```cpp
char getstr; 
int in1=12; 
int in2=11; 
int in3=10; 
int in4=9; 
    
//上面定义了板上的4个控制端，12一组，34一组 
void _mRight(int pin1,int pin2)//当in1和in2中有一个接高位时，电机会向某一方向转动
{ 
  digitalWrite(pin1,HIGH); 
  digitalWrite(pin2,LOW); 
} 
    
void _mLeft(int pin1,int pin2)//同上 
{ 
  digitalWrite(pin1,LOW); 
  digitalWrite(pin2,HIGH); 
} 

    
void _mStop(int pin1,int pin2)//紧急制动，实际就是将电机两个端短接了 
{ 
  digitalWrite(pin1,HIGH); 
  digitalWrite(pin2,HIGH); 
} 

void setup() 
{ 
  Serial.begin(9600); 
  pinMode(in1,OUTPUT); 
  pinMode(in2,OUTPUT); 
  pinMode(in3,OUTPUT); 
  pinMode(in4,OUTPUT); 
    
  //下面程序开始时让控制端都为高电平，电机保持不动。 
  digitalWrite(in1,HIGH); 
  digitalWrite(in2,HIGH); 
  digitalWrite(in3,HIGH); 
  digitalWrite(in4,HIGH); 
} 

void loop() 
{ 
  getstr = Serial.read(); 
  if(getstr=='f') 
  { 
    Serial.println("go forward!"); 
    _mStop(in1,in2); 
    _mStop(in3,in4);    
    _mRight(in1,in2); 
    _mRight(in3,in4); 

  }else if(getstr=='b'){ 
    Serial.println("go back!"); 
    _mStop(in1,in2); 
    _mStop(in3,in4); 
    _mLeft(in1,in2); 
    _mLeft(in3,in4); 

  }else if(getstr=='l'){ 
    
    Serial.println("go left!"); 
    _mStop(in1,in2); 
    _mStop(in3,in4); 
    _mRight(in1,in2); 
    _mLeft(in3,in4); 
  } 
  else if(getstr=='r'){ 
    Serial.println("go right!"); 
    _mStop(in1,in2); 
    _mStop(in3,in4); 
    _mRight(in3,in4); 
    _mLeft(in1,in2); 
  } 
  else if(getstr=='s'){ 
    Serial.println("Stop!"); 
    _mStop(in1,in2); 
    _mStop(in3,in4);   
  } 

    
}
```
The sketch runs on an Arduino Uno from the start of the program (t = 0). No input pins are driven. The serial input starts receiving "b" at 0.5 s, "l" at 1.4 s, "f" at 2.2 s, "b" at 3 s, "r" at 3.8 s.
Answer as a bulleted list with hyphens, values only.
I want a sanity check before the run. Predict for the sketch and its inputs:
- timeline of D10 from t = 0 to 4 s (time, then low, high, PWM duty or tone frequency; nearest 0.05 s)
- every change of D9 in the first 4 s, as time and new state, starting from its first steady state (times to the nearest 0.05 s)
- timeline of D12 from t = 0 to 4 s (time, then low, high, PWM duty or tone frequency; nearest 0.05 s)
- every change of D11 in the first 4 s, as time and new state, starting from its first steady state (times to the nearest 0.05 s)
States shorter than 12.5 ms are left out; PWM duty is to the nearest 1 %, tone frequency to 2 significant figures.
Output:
- 0 s high; 0.5 s low; 2.2 s high; 3 s low; 3.8 s high
- 0 s high; 2.2 s low; 3 s high; 3.8 s low
- 0 s high; 0.5 s low; 1.4 s high; 3 s low
- 0 s high; 1.4 s low; 3 s high
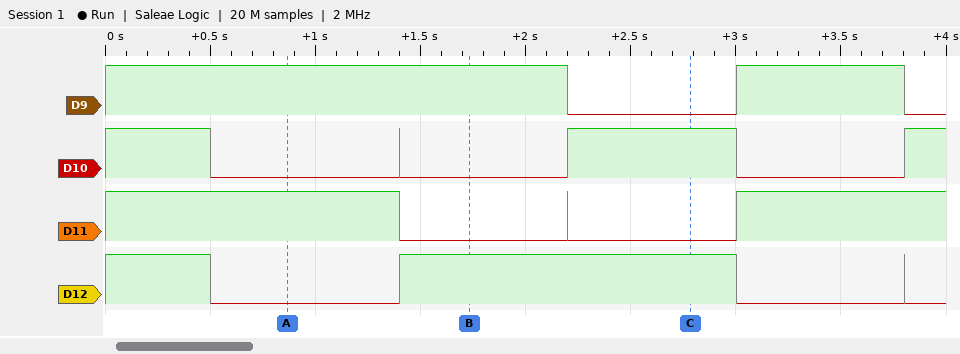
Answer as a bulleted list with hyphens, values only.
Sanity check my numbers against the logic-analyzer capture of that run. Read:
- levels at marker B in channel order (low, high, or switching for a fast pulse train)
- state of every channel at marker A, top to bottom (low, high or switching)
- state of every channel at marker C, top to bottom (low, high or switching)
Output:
- D9 high, D10 low, D11 low, D12 high
- D9 high, D10 low, D11 high, D12 low
- D9 low, D10 high, D11 low, D12 high
